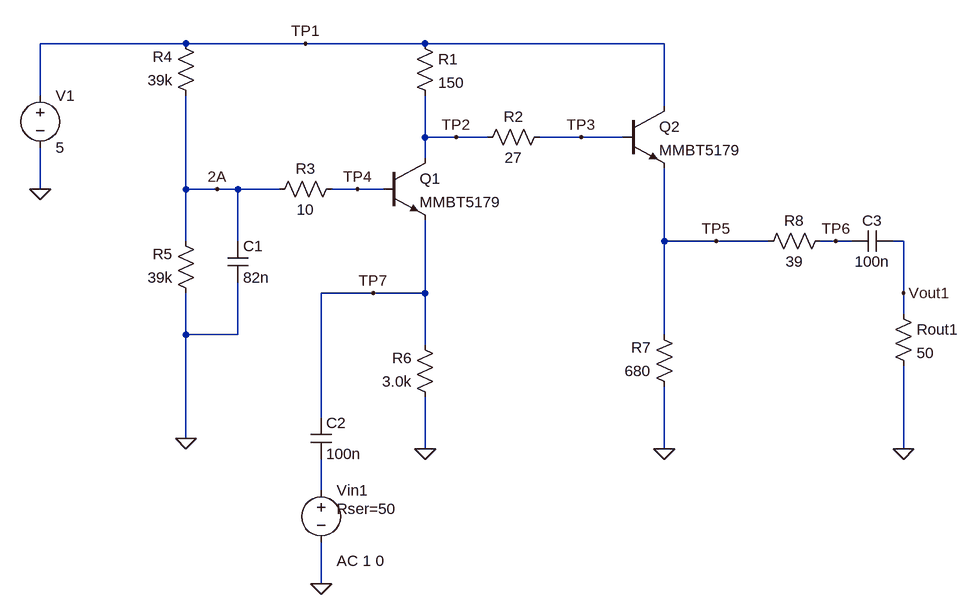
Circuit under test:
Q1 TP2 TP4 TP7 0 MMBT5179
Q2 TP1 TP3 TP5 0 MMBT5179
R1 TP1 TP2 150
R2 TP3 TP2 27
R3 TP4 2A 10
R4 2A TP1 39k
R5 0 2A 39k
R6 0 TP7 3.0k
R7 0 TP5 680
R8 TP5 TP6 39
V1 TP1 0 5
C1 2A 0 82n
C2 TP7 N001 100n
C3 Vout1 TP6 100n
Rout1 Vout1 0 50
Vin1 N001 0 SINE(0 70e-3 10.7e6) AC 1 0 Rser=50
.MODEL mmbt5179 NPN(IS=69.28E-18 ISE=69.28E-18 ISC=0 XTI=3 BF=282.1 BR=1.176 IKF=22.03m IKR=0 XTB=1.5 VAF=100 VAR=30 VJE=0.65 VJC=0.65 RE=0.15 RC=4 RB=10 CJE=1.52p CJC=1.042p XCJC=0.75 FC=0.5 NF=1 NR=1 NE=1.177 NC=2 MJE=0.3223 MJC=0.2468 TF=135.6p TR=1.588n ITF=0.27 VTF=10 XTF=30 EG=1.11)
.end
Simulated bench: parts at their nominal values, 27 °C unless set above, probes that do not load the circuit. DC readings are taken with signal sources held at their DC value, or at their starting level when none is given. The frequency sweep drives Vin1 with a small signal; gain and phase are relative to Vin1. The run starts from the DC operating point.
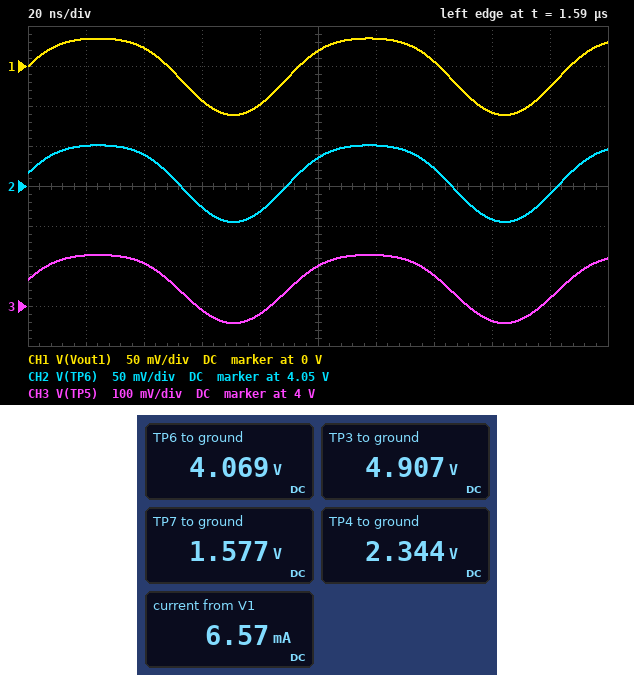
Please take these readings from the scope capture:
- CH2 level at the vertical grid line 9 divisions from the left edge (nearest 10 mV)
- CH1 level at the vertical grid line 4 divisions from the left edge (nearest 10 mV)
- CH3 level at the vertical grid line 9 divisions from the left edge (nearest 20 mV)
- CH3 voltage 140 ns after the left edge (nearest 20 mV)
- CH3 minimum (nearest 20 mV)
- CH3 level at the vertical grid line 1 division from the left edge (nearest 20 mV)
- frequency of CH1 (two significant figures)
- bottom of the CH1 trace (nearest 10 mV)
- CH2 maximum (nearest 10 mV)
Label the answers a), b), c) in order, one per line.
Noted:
a) 4.04 V
b) -50 mV
c) 4.02 V
d) 4.08 V
e) 3.96 V
f) 4.12 V
g) 11 MHz
h) -60 mV
i) 4.10 V
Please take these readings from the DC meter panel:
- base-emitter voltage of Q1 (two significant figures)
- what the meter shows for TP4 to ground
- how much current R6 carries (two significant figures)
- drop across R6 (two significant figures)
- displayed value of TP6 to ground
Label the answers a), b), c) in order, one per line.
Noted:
a) 770 mV
b) 2.344 V
c) 530 µA
d) 1.6 V
e) 4.069 V
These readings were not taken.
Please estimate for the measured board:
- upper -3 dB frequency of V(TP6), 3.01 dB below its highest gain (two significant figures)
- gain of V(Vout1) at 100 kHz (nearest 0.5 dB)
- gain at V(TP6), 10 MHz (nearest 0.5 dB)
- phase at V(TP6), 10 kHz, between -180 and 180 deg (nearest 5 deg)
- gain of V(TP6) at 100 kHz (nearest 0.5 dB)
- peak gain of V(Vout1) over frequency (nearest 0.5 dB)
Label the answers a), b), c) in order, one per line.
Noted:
a) 160 MHz
b) -3.0 dB
c) -2.5 dB
d) 45 deg
e) -2.5 dB
f) -2.5 dB
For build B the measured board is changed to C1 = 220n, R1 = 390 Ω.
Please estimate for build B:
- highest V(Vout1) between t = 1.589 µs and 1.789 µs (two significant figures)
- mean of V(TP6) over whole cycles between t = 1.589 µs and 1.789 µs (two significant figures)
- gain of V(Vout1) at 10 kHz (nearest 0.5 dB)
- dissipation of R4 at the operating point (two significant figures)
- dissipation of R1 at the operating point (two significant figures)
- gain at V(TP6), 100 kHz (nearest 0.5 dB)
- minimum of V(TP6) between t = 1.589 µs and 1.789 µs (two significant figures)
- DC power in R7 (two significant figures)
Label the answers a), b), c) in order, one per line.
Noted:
a) 85 mV
b) 3.9 V
c) -5.5 dB
d) 180 µW
e) 140 µW
f) 5.5 dB
g) 3.8 V
h) 23 mW
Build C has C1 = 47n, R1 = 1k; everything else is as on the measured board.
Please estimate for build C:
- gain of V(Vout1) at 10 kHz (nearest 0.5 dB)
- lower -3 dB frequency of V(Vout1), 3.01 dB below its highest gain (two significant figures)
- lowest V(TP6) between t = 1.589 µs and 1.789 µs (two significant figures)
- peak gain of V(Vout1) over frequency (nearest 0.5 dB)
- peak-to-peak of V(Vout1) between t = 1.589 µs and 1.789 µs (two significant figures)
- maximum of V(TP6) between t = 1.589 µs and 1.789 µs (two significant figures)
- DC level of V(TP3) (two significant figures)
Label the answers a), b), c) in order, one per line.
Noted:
a) 2.0 dB
b) 24 kHz
c) 3.3 V
d) 12.5 dB
e) 430 mV
f) 3.8 V
g) 4.4 V
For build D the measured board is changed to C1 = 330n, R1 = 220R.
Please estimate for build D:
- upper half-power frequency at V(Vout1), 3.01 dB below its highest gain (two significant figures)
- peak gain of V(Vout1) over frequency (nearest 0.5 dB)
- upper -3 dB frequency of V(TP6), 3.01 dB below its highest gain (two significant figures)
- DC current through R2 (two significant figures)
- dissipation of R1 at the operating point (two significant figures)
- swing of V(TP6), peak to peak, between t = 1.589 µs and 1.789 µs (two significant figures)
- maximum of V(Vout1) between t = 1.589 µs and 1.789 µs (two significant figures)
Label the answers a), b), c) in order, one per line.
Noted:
a) 160 MHz
b) 0.5 dB
c) 120 MHz
d) 86 µA
e) 80 µW
f) 140 mV
g) 50 mV
